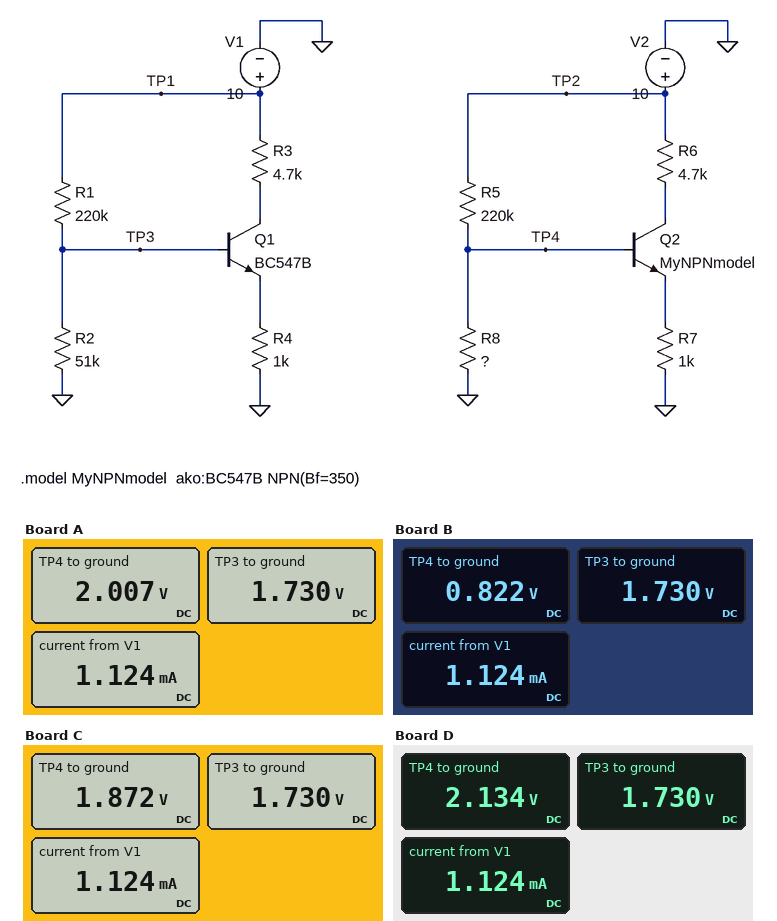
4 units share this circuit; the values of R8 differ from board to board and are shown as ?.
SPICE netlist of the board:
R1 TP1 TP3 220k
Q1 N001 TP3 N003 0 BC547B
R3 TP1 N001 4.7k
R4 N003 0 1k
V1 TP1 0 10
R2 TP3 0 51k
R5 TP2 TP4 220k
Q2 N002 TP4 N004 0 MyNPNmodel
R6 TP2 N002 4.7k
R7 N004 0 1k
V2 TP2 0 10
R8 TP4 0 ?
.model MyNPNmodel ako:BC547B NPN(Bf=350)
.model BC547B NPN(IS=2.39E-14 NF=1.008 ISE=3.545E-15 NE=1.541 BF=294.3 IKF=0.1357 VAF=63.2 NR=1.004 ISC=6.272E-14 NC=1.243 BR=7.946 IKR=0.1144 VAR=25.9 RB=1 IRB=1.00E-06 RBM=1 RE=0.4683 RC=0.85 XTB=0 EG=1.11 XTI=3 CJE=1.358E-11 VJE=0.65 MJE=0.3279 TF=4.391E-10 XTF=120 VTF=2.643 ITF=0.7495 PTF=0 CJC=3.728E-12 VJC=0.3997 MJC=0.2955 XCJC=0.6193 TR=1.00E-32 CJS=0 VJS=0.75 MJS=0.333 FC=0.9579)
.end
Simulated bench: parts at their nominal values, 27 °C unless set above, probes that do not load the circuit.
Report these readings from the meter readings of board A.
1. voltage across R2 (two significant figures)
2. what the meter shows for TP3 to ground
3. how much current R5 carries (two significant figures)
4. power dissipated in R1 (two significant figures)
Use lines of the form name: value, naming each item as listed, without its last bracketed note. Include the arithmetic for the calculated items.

voltage across R2: 1.73 V = 1.7 V
what the meter shows for TP3 to ground: 1.730 V
how much current R5 carries: (10 V - 2.007 V) / 220 kΩ = 36 µA
power dissipated in R1: (10 V - 1.73 V)^2 / 220 kΩ = 310 µW
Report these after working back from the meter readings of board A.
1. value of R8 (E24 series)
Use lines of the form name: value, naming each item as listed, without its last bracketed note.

value of R8: 62 kΩ
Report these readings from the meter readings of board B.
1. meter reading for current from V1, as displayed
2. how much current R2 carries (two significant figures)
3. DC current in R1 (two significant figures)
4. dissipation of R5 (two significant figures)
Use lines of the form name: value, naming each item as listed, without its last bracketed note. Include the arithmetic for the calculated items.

meter reading for current from V1, as displayed: 1.124 mA
how much current R2 carries: (1.73 V) / 51 kΩ = 34 µA
DC current in R1: (10 V - 1.73 V) / 220 kΩ = 38 µA
dissipation of R5: (10 V - 822 mV)^2 / 220 kΩ = 380 µW
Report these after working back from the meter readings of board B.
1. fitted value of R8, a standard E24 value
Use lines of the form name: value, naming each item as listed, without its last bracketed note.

fitted value of R8, a standard E24 value: 20 kΩ
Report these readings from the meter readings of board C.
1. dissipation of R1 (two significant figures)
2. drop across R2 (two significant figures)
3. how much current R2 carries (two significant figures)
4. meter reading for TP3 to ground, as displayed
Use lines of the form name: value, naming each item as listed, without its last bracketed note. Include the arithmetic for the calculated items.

dissipation of R1: (10 V - 1.73 V)^2 / 220 kΩ = 310 µW
drop across R2: 1.73 V = 1.7 V
how much current R2 carries: (1.73 V) / 51 kΩ = 34 µA
meter reading for TP3 to ground, as displayed: 1.730 V
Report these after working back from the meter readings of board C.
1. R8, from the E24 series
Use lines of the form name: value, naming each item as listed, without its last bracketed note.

R8, from the E24 series: 56 kΩ
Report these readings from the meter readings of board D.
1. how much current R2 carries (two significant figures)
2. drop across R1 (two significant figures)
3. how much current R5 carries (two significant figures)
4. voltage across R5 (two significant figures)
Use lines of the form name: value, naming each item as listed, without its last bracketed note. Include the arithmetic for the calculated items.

how much current R2 carries: (1.73 V) / 51 kΩ = 34 µA
drop across R1: 10 V - 1.73 V = 8.3 V
how much current R5 carries: (10 V - 2.134 V) / 220 kΩ = 36 µA
voltage across R5: 10 V - 2.134 V = 7.9 V
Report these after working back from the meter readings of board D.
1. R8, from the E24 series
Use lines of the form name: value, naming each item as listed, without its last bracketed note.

R8, from the E24 series: 68 kΩ
